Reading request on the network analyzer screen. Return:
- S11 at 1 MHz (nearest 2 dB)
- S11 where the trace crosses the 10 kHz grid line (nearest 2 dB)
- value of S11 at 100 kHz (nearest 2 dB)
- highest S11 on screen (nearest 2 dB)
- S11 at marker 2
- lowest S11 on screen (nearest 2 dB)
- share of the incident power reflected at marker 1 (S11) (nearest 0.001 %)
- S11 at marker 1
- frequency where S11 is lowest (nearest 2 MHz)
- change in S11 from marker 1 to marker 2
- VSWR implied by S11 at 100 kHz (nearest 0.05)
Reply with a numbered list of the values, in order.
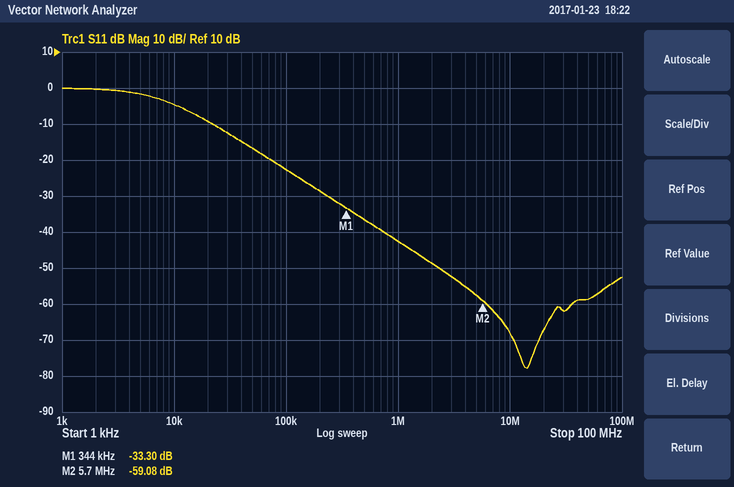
1. -42 dB
2. -4 dB
3. -22 dB
4. 0 dB
5. -59.08 dB
6. -78 dB
7. 0.047 %
8. -33.30 dB
9. 14 MHz
10. -25.78 dB
11. 1.15
